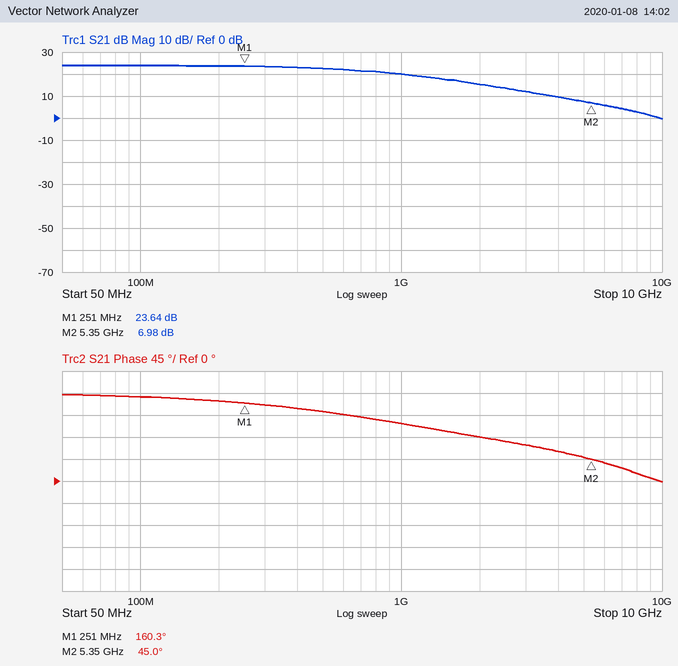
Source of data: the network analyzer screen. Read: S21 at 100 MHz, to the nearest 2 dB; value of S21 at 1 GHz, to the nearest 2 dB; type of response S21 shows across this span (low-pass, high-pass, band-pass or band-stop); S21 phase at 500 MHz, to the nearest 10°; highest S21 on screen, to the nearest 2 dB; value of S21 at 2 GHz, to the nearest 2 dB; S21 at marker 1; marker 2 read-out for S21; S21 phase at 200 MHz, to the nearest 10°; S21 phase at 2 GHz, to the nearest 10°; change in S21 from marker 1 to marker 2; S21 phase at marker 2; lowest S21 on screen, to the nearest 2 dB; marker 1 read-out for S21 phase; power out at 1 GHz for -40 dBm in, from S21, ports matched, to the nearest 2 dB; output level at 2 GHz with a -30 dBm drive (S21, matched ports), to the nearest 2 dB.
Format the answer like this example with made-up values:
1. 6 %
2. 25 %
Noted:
1. 24 dB
2. 20 dB
3. low-pass
4. 140°
5. 24 dB
6. 16 dB
7. 23.64 dB
8. 6.98 dB
9. 160°
10. 90°
11. -16.66 dB
12. 45.0°
13. 0 dB
14. 160.3°
15. -20 dBm
16. -14 dBm
